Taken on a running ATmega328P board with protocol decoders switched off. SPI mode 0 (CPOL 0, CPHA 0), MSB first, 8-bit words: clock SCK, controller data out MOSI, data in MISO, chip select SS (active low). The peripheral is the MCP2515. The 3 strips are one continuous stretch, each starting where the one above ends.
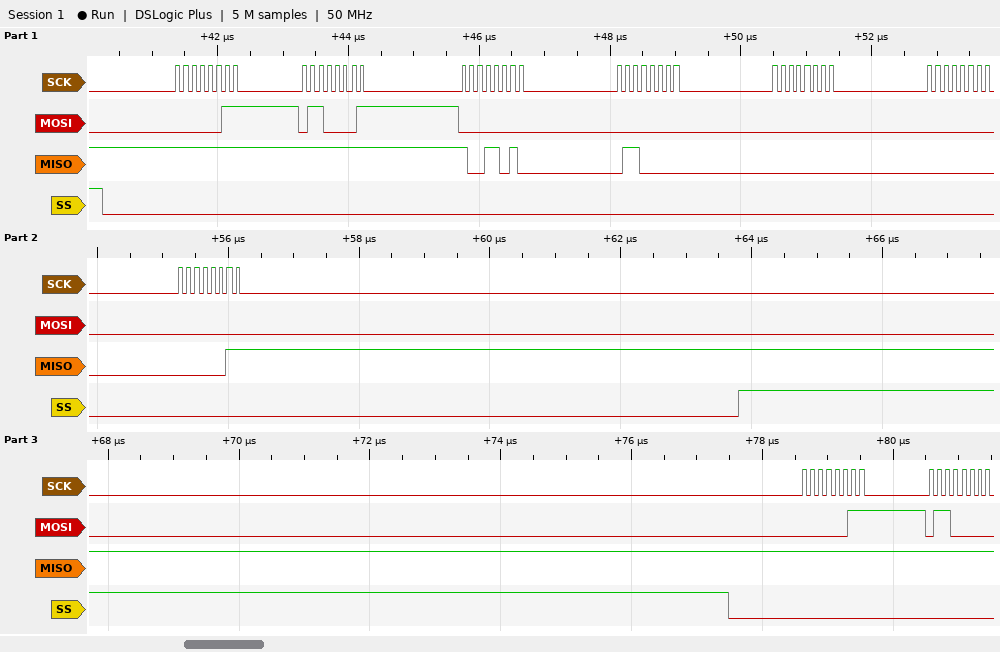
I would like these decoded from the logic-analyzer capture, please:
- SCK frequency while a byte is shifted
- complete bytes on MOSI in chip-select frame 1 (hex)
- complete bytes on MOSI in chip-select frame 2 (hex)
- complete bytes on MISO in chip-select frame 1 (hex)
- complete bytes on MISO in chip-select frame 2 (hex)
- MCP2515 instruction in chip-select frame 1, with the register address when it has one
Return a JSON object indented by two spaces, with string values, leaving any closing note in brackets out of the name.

{
  "SCK frequency while a byte is shifted": "8 MHz",
  "complete bytes on MOSI in chip-select frame 1": "0x03 0x61 0x00 0x00 0x00 0x00 0x00",
  "complete bytes on MOSI in chip-select frame 2": "0x03 0x60",
  "complete bytes on MISO in chip-select frame 1": "0xFF 0xFF 0x9A 0x60 0x00 0x00 0x03",
  "complete bytes on MISO in chip-select frame 2": "0xFF 0xFF",
  "MCP2515 instruction in chip-select frame 1, with the register address when it has one": "READ 0x61"
}
